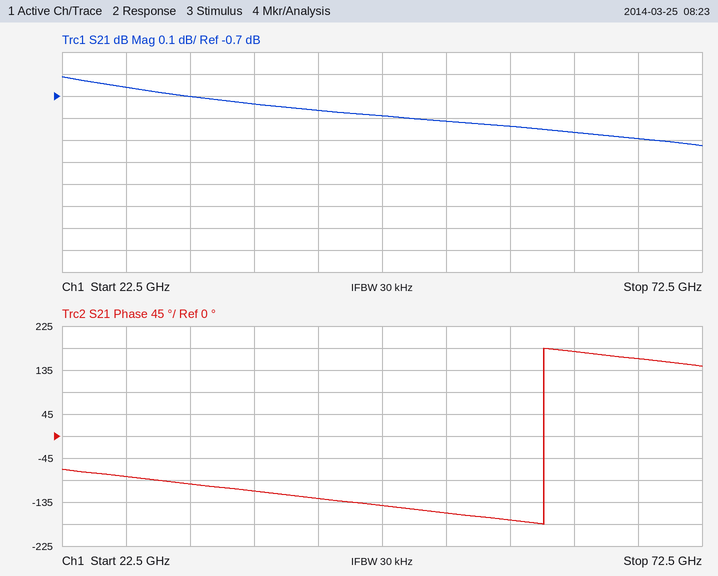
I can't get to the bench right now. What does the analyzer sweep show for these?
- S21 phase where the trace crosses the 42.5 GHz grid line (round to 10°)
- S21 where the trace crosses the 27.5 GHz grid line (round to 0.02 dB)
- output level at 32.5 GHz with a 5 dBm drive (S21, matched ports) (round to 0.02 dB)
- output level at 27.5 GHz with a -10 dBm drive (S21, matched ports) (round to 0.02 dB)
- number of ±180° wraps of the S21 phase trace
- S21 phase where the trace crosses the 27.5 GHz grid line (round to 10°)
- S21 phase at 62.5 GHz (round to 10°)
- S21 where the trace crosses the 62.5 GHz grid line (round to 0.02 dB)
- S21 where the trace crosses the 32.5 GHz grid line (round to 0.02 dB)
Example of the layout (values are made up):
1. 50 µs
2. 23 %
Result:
1. -130°
2. -0.66 dB
3. 4.30 dBm
4. -10.66 dBm
5. 1
6. -80°
7. 170°
8. -0.86 dB
9. -0.70 dB
